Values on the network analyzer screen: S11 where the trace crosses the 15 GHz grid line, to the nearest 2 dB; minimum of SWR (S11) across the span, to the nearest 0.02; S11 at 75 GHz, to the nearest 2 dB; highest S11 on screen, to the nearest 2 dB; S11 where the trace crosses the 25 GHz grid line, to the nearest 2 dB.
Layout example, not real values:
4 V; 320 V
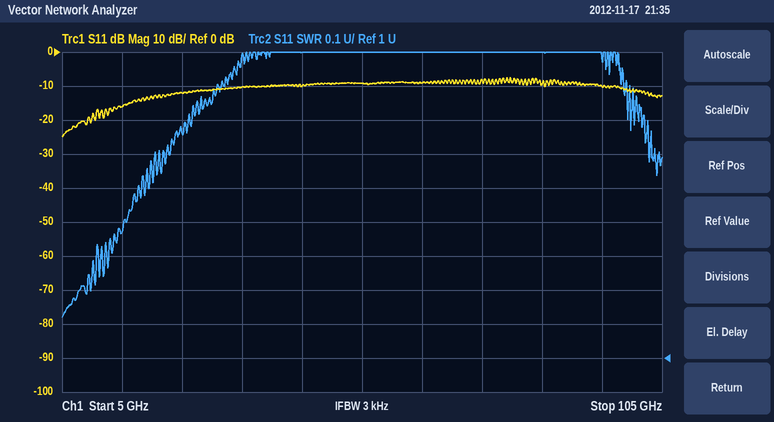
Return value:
-16 dB; 1.12; -8 dB; -8 dB; -12 dB
